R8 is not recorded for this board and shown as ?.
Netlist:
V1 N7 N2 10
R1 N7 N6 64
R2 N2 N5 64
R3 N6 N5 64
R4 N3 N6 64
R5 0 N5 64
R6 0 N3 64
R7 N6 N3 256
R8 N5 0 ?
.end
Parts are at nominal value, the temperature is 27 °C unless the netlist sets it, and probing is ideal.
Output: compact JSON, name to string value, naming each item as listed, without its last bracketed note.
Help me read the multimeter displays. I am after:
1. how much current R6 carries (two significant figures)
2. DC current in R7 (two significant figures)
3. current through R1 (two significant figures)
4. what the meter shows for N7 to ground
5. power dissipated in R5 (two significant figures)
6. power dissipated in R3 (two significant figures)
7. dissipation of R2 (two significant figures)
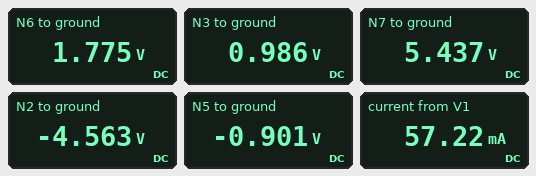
{"how much current R6 carries": "15 mA", "DC current in R7": "3.1 mA", "current through R1": "57 mA", "what the meter shows for N7 to ground": "5.437 V", "power dissipated in R5": "13 mW", "power dissipated in R3": "110 mW", "dissipation of R2": "210 mW"}
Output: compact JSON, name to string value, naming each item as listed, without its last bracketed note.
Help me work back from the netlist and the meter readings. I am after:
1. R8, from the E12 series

{"R8, from the E12 series": "680 Ω"}
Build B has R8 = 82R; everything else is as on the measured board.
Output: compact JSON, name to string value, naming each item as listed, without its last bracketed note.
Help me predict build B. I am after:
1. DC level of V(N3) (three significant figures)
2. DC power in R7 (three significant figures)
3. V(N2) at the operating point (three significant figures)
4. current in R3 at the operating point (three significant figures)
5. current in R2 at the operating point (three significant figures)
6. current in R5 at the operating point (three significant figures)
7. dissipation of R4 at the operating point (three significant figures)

{"DC level of V(N3)": "1.10 V", "DC power in R7": "3.03 mW", "V(N2) at the operating point": "-4.32 V", "current in R3 at the operating point": "40.6 mA", "current in R2 at the operating point": "57.8 mA", "current in R5 at the operating point": "9.66 mA", "dissipation of R4 at the operating point": "12.1 mW"}
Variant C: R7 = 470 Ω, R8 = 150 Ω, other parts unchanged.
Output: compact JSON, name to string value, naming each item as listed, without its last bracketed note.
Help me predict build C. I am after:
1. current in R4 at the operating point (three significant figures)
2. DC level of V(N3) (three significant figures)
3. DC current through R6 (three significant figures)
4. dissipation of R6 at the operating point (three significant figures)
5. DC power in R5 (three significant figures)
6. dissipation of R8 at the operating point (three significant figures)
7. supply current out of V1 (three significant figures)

{"current in R4 at the operating point": "14.1 mA", "DC level of V(N3)": "1.03 V", "DC current through R6": "16.0 mA", "dissipation of R6 at the operating point": "16.5 mW", "DC power in R5": "8.09 mW", "dissipation of R8 at the operating point": "3.45 mW", "supply current out of V1": "57.4 mA"}
